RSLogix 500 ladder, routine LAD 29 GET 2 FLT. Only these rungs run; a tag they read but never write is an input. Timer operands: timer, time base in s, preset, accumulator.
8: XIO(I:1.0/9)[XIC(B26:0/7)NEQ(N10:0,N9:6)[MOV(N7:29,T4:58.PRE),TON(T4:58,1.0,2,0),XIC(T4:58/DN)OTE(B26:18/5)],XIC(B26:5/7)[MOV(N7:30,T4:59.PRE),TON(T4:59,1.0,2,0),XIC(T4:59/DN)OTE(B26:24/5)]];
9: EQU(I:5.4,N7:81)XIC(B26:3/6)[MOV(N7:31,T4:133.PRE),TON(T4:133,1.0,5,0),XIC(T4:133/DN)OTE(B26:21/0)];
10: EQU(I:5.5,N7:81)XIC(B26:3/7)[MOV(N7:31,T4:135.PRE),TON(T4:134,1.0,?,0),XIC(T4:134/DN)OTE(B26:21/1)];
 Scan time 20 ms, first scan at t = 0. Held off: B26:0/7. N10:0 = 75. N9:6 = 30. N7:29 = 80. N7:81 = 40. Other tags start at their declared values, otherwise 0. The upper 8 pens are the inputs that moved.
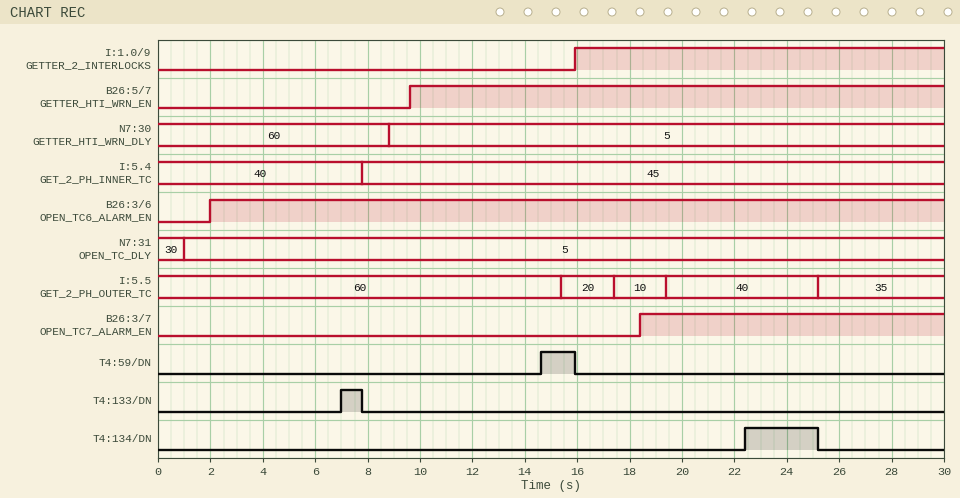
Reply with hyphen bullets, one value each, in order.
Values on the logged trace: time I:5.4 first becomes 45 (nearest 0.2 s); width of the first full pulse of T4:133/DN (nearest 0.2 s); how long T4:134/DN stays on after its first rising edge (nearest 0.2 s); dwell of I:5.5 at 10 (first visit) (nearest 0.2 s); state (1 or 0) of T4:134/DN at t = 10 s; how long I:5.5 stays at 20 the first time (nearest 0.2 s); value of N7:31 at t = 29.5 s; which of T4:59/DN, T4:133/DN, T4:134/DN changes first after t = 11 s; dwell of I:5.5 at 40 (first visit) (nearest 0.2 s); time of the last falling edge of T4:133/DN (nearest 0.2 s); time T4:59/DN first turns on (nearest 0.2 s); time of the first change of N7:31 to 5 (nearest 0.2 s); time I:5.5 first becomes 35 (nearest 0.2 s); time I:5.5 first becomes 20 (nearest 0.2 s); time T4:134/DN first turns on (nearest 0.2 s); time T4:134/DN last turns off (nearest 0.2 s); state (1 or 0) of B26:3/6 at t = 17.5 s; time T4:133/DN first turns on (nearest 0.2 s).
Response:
- 7.8 s
- 0.8 s
- 2.8 s
- 2.0 s
- 0
- 2.0 s
- 5
- T4:59/DN
- 5.8 s
- 7.8 s
- 14.6 s
- 1.0 s
- 25.2 s
- 15.4 s
- 22.4 s
- 25.2 s
- 1
- 7.0 s
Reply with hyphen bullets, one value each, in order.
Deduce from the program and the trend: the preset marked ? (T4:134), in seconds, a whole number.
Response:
- 3 s
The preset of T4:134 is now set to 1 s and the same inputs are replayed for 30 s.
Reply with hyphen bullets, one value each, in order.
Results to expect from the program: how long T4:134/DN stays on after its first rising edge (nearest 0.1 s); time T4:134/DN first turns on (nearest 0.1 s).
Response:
- 4.8 s
- 20.4 s
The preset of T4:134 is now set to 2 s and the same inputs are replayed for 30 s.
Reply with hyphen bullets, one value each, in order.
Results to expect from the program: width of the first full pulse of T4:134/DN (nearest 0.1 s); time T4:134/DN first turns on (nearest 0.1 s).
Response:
- 3.8 s
- 21.4 s
